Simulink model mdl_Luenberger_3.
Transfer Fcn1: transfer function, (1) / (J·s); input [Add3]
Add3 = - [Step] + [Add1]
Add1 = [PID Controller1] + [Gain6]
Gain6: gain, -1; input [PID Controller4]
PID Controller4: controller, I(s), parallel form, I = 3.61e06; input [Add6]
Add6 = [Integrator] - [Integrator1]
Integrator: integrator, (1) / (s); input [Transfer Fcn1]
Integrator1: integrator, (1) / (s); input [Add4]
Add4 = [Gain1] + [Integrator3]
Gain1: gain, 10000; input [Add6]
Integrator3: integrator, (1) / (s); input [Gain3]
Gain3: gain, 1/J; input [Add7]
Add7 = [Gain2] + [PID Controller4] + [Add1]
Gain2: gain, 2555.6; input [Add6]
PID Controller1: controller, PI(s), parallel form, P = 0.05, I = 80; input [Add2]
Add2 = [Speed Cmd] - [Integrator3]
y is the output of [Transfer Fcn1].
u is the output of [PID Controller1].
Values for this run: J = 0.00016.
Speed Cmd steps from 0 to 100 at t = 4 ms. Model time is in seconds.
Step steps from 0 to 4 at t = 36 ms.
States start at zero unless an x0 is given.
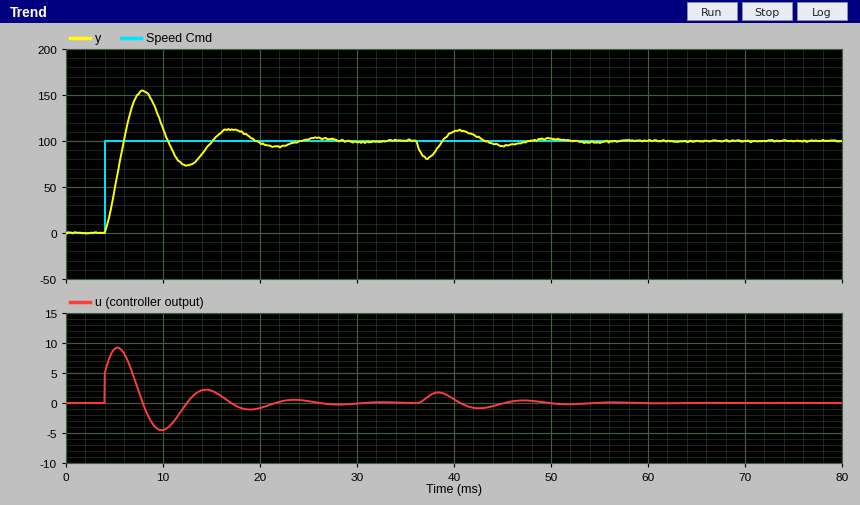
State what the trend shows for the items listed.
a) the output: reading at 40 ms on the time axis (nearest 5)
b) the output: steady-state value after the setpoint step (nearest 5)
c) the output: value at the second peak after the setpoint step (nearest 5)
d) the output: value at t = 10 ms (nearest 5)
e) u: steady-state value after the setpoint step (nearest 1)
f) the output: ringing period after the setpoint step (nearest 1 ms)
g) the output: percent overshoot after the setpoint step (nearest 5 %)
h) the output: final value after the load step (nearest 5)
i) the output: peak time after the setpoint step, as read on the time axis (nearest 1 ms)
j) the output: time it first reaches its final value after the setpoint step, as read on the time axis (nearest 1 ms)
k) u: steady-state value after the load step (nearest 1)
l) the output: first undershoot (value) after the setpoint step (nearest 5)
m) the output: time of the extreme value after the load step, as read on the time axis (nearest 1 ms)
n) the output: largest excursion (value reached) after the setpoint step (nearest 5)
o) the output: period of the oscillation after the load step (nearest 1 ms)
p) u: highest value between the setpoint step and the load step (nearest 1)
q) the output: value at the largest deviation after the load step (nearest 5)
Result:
110
100
115
115
0
9 ms
55 %
100
8 ms
6 ms
0
75
37 ms
155
8 ms
9
80
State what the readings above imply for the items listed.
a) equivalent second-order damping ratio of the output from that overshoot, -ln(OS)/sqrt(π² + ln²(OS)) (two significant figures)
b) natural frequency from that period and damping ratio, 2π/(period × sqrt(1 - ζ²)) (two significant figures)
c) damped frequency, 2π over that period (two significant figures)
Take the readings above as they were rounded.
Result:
0.19
0.71 rad/ms
0.70 rad/ms
